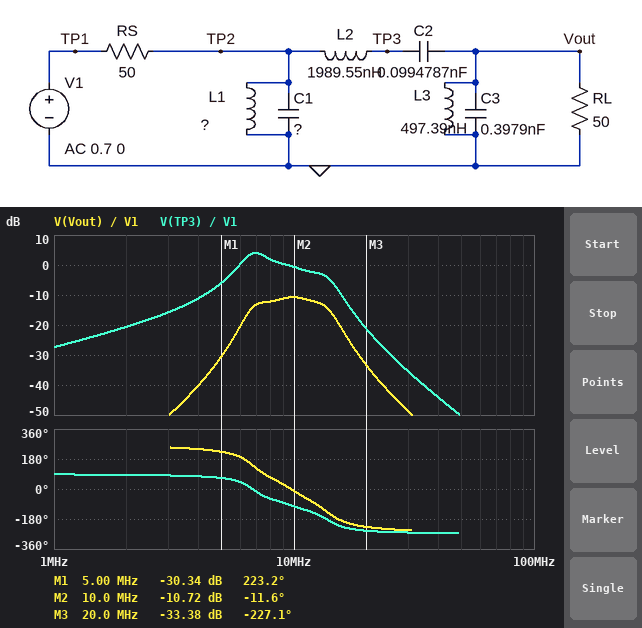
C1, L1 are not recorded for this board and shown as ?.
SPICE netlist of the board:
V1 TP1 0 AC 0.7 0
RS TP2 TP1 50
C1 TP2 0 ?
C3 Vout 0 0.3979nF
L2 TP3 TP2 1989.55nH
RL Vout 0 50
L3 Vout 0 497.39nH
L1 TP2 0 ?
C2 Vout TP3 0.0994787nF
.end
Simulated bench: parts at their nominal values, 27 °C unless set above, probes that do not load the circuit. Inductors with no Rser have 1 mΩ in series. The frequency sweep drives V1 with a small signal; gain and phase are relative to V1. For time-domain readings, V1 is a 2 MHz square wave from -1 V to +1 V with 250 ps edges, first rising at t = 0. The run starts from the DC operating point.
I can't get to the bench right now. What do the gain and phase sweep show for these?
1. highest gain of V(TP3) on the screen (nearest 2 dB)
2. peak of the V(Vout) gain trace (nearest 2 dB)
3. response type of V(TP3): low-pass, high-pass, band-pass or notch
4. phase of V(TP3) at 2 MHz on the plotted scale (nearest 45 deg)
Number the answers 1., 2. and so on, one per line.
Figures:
1. 4 dB
2. -10 dB
3. band-pass
4. 90 deg
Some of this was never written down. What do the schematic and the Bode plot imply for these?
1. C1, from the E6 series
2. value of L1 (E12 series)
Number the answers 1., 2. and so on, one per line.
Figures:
1. 1.5 nF
2. 330 nH
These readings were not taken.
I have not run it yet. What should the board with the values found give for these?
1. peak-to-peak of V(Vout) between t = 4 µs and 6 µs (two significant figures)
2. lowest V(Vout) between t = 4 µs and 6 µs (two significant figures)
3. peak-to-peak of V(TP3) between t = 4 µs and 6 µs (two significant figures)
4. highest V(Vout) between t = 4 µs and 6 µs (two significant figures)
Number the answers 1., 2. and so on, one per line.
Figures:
1. 280 mV
2. -140 mV
3. 1.4 V
4. 140 mV
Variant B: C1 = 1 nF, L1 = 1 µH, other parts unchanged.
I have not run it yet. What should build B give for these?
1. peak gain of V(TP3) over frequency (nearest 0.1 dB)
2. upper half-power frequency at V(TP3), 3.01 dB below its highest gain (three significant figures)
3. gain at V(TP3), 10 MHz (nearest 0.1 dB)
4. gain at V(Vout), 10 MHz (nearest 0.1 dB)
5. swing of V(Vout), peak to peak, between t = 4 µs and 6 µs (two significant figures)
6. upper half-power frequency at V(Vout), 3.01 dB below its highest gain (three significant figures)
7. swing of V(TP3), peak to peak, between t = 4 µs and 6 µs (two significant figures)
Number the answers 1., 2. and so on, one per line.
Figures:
1. 1.8 dB
2. 11.0 MHz
3. -0.7 dB
4. -10.8 dB
5. 330 mV
6. 14.3 MHz
7. 2.4 V
